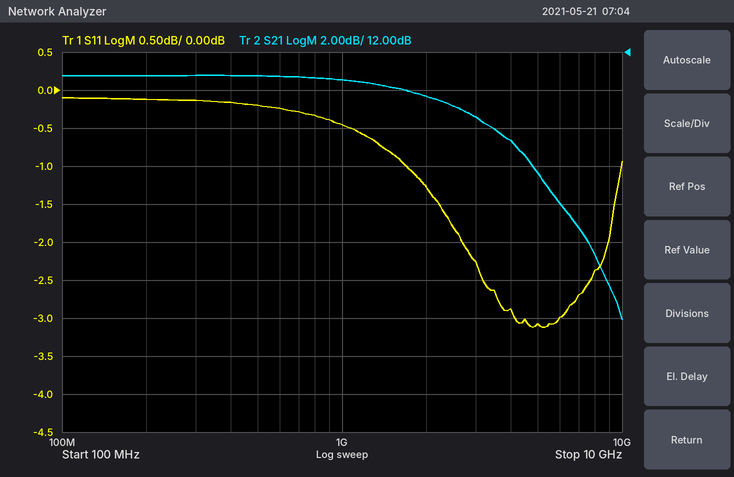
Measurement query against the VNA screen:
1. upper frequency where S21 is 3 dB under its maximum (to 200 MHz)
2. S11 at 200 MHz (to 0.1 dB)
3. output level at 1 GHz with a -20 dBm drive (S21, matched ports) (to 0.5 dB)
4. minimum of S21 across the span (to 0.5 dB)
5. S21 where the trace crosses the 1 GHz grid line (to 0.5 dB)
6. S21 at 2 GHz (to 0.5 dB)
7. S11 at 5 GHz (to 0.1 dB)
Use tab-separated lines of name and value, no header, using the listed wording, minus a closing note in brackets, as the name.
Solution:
upper frequency where S21 is 3 dB under its maximum	3.6 GHz
S11 at 200 MHz	-0.1 dB
output level at 1 GHz with a -20 dBm drive (S21, matched ports)	-9.5 dBm
minimum of S21 across the span	-2.0 dB
S21 where the trace crosses the 1 GHz grid line	10.5 dB
S21 at 2 GHz	9.5 dB
S11 at 5 GHz	-3.1 dB
